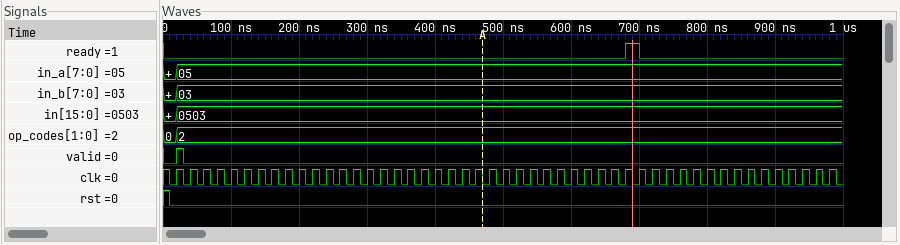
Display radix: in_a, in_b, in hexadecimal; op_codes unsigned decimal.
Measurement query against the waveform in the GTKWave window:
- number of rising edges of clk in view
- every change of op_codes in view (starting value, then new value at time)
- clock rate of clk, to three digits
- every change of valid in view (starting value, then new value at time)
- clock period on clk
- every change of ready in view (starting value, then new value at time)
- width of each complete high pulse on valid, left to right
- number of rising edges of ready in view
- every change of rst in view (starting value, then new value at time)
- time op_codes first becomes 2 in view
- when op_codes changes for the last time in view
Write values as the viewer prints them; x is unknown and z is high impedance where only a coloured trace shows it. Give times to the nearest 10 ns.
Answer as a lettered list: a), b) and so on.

a) 49
b) 0, 2 at 20 ns
c) 50.0 MHz
d) 0, 1 at 20 ns, 0 at 30 ns
e) 20 ns
f) 0, 1 at 680 ns, 0 at 700 ns
g) 10 ns
h) 1
i) 1, 0 at 10 ns
j) 20 ns
k) 20 ns
